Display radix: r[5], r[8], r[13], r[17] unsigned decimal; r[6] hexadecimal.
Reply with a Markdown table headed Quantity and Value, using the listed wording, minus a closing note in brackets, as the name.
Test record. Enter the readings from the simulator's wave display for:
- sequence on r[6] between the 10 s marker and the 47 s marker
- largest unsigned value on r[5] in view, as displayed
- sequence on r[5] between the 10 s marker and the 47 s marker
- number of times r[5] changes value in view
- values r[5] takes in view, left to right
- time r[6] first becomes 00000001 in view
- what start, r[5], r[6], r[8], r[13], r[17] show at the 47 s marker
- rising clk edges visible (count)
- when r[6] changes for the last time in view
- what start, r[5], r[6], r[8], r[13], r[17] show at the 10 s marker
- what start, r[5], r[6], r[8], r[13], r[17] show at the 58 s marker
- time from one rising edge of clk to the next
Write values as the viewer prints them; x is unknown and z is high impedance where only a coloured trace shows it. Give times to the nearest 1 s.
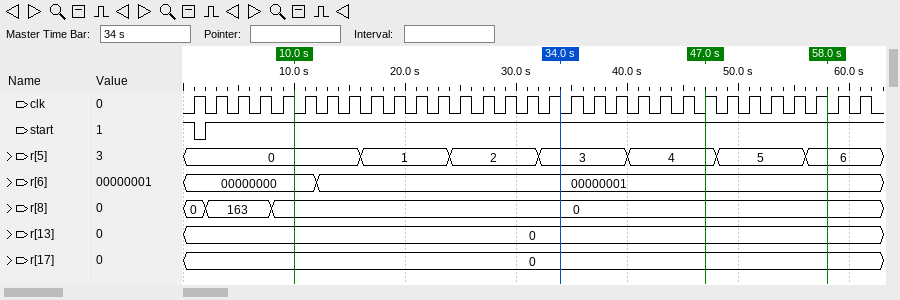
| Quantity | Value |
|---|---|
| sequence on r[6] between the 10 s marker and the 47 s marker | 00000000, 00000001 |
| largest unsigned value on r[5] in view, as displayed | 6 |
| sequence on r[5] between the 10 s marker and the 47 s marker | 0, 1, 2, 3, 4 |
| number of times r[5] changes value in view | 6 |
| values r[5] takes in view, left to right | 0, 1, 2, 3, 4, 5, 6 |
| time r[6] first becomes 00000001 in view | 12 s |
| what start, r[5], r[6], r[8], r[13], r[17] show at the 47 s marker | start=1, r[5]=4, r[6]=00000001, r[8]=0, r[13]=0, r[17]=0 |
| rising clk edges visible | 31 |
| when r[6] changes for the last time in view | 12 s |
| what start, r[5], r[6], r[8], r[13], r[17] show at the 10 s marker | start=1, r[5]=0, r[6]=00000000, r[8]=0, r[13]=0, r[17]=0 |
| what start, r[5], r[6], r[8], r[13], r[17] show at the 58 s marker | start=1, r[5]=6, r[6]=00000001, r[8]=0, r[13]=0, r[17]=0 |
| time from one rising edge of clk to the next | 2 s |
